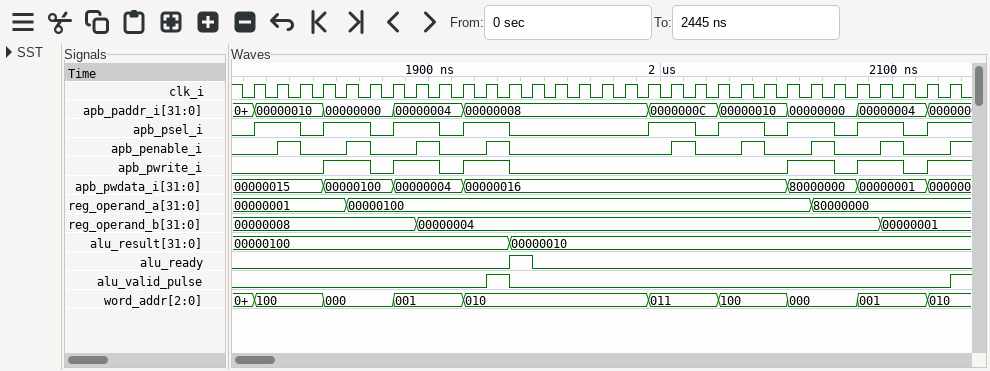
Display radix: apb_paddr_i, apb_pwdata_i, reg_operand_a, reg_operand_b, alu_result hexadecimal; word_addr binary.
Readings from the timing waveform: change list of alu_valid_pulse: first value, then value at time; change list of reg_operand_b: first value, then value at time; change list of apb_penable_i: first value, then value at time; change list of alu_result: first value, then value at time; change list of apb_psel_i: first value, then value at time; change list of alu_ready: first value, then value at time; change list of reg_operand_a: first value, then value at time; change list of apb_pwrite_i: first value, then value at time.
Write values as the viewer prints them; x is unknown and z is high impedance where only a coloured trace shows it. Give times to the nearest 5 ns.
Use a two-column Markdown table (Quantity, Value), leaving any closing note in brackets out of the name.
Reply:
| Quantity | Value |
|---|---|
| change list of alu_valid_pulse: first value, then value at time | 0, 1 at 1925 ns, 0 at 1935 ns, 1 at 2125 ns |
| change list of reg_operand_b: first value, then value at time | 00000008, 00000004 at 1895 ns, 00000001 at 2095 ns |
| change list of apb_penable_i: first value, then value at time | 0, 1 at 1835 ns, 0 at 1845 ns, 1 at 1865 ns, 0 at 1875 ns, 1 at 1895 ns, 0 at 1905 ns, 1 at 1925 ns, 0 at 1935 ns, 1 at 2005 ns, 0 at 2015 ns, 1 at 2035 ns, 0 at 2045 ns, 1 at 2065 ns, 0 at 2075 ns, 1 at 2095 ns, 0 at 2105 ns, 1 at 2125 ns |
| change list of alu_result: first value, then value at time | 00000100, 00000010 at 1935 ns |
| change list of apb_psel_i: first value, then value at time | 0, 1 at 1825 ns, 0 at 1845 ns, 1 at 1855 ns, 0 at 1875 ns, 1 at 1885 ns, 0 at 1905 ns, 1 at 1915 ns, 0 at 1935 ns, 1 at 1995 ns, 0 at 2015 ns, 1 at 2025 ns, 0 at 2045 ns, 1 at 2055 ns, 0 at 2075 ns, 1 at 2085 ns, 0 at 2105 ns, 1 at 2115 ns |
| change list of alu_ready: first value, then value at time | 0, 1 at 1935 ns, 0 at 1945 ns |
| change list of reg_operand_a: first value, then value at time | 00000001, 00000100 at 1865 ns, 80000000 at 2065 ns |
| change list of apb_pwrite_i: first value, then value at time | 0, 1 at 1855 ns, 0 at 1875 ns, 1 at 1885 ns, 0 at 1905 ns, 1 at 1915 ns, 0 at 1935 ns, 1 at 2055 ns, 0 at 2075 ns, 1 at 2085 ns, 0 at 2105 ns, 1 at 2115 ns |
